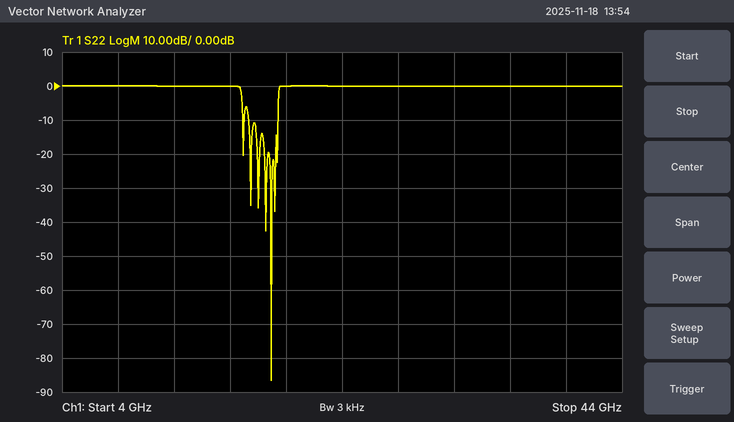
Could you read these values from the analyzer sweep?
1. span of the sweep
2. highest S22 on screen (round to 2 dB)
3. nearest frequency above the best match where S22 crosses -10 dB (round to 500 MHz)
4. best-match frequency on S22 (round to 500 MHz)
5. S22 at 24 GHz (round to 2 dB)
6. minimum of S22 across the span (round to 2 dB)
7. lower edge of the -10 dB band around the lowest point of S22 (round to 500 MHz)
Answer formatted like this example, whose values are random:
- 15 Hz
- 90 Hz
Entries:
- 40 GHz
- 0 dB
- 19.5 GHz
- 19.0 GHz
- 0 dB
- -86 dB
- 17.5 GHz
